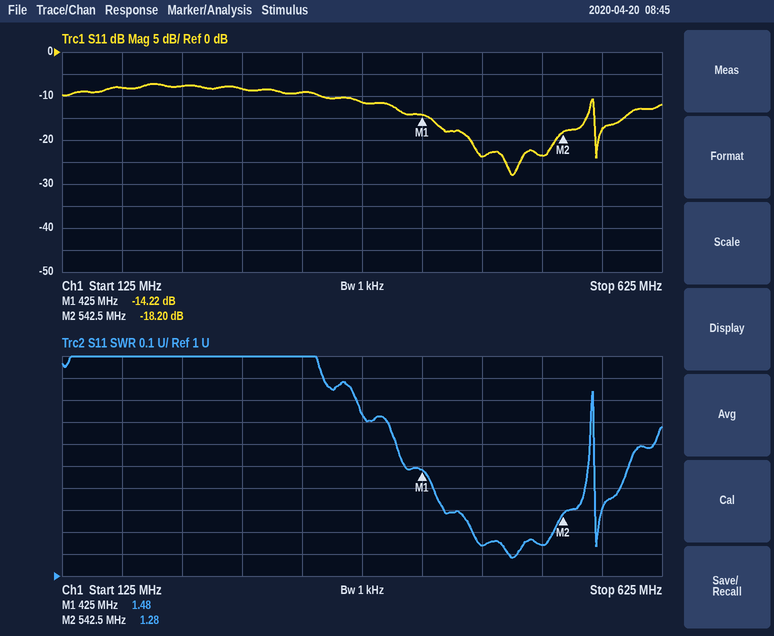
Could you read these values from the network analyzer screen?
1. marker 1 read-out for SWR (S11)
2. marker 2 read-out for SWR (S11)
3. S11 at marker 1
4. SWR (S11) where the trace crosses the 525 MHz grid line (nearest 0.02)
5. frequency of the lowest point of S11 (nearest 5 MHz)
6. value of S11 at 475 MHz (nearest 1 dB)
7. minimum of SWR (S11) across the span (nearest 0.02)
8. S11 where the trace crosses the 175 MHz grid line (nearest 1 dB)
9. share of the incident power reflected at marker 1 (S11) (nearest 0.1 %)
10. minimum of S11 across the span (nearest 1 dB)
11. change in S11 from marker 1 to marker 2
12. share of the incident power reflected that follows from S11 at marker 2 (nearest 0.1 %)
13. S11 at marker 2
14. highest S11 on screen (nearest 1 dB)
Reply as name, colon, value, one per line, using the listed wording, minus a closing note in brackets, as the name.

marker 1 read-out for SWR: 1.48
marker 2 read-out for SWR: 1.28
S11 at marker 1: -14.22 dB
SWR (S11) where the trace crosses the 525 MHz grid line: 1.14
frequency of the lowest point of S11: 500 MHz
value of S11 at 475 MHz: -24 dB
minimum of SWR (S11) across the span: 1.08
S11 where the trace crosses the 175 MHz grid line: -8 dB
share of the incident power reflected at marker 1 (S11): 3.8 %
minimum of S11 across the span: -28 dB
change in S11 from marker 1 to marker 2: -3.98 dB
share of the incident power reflected that follows from S11 at marker 2: 1.5 %
S11 at marker 2: -18.20 dB
highest S11 on screen: -7 dB
